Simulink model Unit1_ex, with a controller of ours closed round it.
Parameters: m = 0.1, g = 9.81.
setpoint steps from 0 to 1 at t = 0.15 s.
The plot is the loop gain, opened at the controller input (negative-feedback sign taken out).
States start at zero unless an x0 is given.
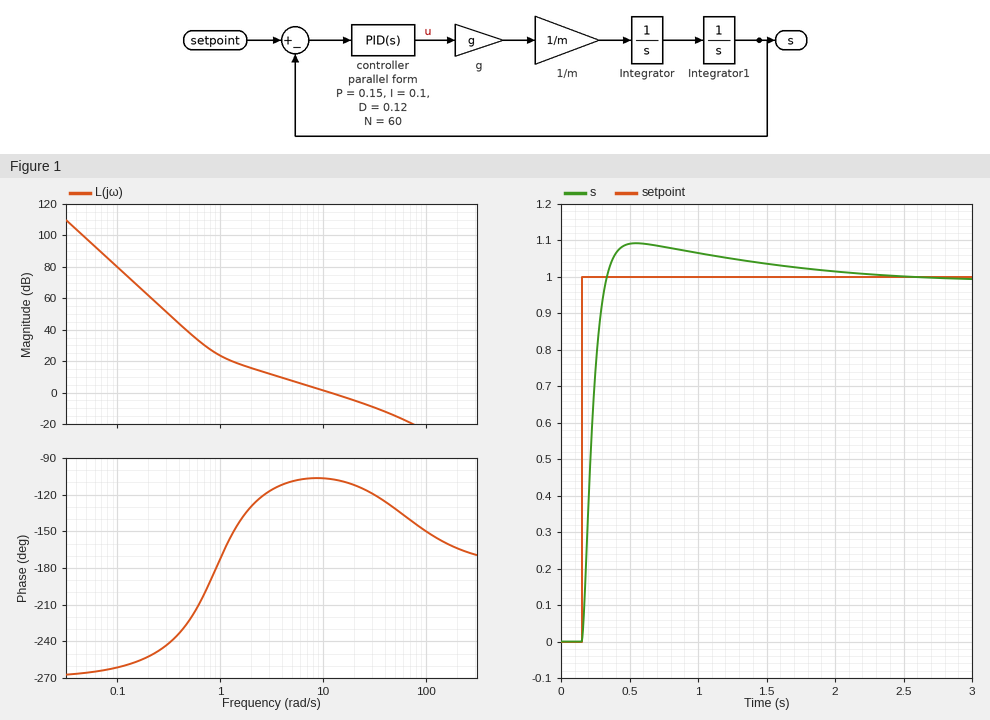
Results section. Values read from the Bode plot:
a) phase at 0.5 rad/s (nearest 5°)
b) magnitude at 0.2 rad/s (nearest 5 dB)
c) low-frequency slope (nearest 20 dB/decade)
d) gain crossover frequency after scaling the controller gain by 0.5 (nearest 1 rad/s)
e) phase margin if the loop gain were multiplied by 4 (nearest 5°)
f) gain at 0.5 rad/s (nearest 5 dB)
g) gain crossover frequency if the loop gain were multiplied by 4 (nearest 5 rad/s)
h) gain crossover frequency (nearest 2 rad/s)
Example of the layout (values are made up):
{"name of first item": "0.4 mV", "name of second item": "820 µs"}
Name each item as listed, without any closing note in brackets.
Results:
{"phase at 0.5 rad/s": "-225°", "magnitude at 0.2 rad/s": "60 dB", "low-frequency slope": "-60 dB/decade", "gain crossover frequency after scaling the controller gain by 0.5": "6 rad/s", "phase margin if the loop gain were multiplied by 4": "55°", "gain at 0.5 rad/s": "40 dB", "gain crossover frequency if the loop gain were multiplied by 4": "40 rad/s", "gain crossover frequency": "12 rad/s"}
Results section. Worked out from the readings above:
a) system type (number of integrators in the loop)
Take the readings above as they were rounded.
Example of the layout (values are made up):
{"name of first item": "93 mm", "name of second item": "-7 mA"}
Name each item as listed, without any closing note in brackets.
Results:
{"system type": "3"}
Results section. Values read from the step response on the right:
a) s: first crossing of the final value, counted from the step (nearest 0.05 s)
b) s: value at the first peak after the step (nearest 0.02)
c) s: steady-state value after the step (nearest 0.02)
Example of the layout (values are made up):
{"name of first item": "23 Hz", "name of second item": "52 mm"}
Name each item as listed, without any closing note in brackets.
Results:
{"s: first crossing of the final value, counted from the step": "0.20 s", "s: value at the first peak after the step": "1.10", "s: steady-state value after the step": "1.00"}
